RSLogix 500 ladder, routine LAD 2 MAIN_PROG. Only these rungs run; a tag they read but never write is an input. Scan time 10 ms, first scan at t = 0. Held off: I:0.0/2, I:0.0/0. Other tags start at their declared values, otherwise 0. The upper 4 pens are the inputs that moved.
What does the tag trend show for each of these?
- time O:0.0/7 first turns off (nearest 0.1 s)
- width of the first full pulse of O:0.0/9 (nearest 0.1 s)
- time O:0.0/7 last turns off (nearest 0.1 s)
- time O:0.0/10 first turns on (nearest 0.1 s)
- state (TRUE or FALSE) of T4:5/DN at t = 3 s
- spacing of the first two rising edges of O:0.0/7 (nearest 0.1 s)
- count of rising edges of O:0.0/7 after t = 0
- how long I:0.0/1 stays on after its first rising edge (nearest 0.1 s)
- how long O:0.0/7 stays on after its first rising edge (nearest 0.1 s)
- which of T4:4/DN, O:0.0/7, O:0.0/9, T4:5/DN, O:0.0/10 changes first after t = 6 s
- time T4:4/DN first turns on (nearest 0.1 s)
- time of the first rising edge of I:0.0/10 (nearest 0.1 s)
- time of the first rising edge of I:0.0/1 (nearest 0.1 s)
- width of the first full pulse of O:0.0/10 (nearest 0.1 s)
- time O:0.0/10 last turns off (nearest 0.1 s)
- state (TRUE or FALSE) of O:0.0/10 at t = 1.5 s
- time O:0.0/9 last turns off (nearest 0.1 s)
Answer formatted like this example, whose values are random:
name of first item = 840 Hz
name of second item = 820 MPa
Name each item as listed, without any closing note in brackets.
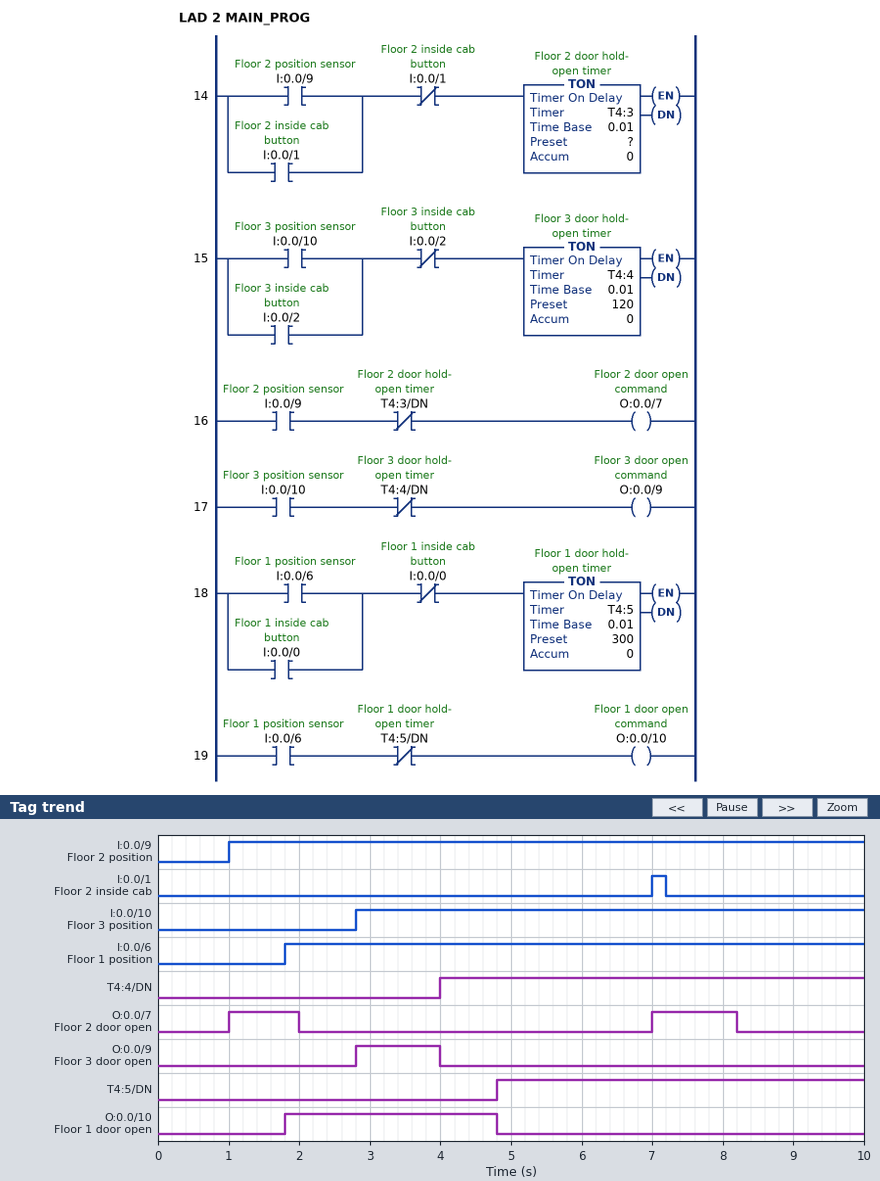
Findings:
time O:0.0/7 first turns off = 2.0 s
width of the first full pulse of O:0.0/9 = 1.2 s
time O:0.0/7 last turns off = 8.2 s
time O:0.0/10 first turns on = 1.8 s
state (TRUE or FALSE) of T4:5/DN at t = 3 s = FALSE
spacing of the first two rising edges of O:0.0/7 = 6.0 s
count of rising edges of O:0.0/7 after t = 0 = 2
how long I:0.0/1 stays on after its first rising edge = 0.2 s
how long O:0.0/7 stays on after its first rising edge = 1.0 s
which of T4:4/DN, O:0.0/7, O:0.0/9, T4:5/DN, O:0.0/10 changes first after t = 6 s = O:0.0/7
time T4:4/DN first turns on = 4.0 s
time of the first rising edge of I:0.0/10 = 2.8 s
time of the first rising edge of I:0.0/1 = 7.0 s
width of the first full pulse of O:0.0/10 = 3.0 s
time O:0.0/10 last turns off = 4.8 s
state (TRUE or FALSE) of O:0.0/10 at t = 1.5 s = FALSE
time O:0.0/9 last turns off = 4.0 s
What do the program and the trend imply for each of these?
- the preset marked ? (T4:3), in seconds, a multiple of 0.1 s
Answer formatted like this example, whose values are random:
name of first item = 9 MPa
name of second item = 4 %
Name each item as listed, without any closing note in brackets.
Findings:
the preset marked ? (T4:3), in seconds, a multiple of 0.1 s = 1.0 s
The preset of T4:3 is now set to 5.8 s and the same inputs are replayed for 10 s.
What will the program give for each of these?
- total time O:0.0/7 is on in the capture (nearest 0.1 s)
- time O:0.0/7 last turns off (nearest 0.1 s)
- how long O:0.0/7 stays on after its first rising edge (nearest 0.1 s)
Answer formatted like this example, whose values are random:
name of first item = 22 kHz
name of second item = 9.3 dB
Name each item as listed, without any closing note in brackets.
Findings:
total time O:0.0/7 is on in the capture = 8.8 s
time O:0.0/7 last turns off = 6.8 s
how long O:0.0/7 stays on after its first rising edge = 5.8 s
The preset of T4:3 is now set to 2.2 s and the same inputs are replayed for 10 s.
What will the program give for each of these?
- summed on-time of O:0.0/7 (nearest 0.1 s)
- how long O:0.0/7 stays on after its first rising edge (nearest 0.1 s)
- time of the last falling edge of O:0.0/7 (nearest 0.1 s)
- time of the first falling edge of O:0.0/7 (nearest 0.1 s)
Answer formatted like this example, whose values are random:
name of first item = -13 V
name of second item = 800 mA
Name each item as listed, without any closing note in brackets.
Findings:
summed on-time of O:0.0/7 = 4.6 s
how long O:0.0/7 stays on after its first rising edge = 2.2 s
time of the last falling edge of O:0.0/7 = 9.4 s
time of the first falling edge of O:0.0/7 = 3.2 s
